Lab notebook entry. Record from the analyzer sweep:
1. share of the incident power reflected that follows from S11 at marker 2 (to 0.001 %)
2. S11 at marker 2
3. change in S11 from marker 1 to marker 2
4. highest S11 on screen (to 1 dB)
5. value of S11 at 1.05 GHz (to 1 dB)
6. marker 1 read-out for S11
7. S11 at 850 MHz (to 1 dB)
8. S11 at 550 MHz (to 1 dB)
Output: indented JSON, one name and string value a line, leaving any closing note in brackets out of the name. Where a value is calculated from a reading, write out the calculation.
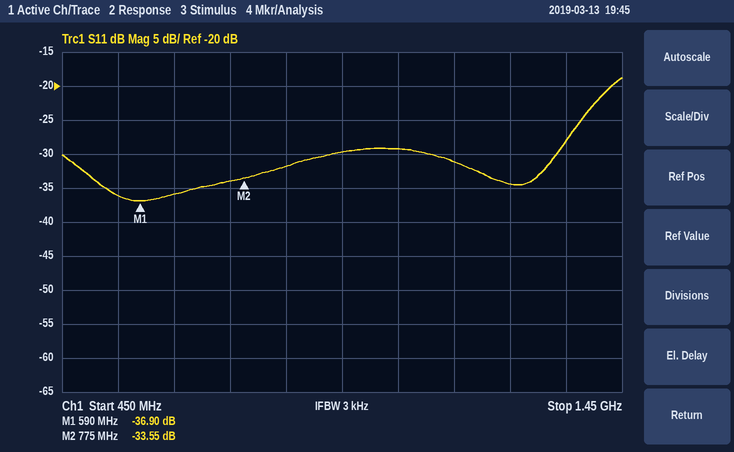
{
  "share of the incident power reflected that follows from S11 at marker 2": "10^(-33.55/10) ≈ 0.044 %",
  "S11 at marker 2": "-33.55 dB",
  "change in S11 from marker 1 to marker 2": "-33.55 − (-36.9) = 3.35 dB",
  "highest S11 on screen": "-19 dB",
  "value of S11 at 1.05 GHz": "-29 dB",
  "marker 1 read-out for S11": "-36.90 dB",
  "S11 at 850 MHz": "-32 dB",
  "S11 at 550 MHz": "-36 dB"
}
